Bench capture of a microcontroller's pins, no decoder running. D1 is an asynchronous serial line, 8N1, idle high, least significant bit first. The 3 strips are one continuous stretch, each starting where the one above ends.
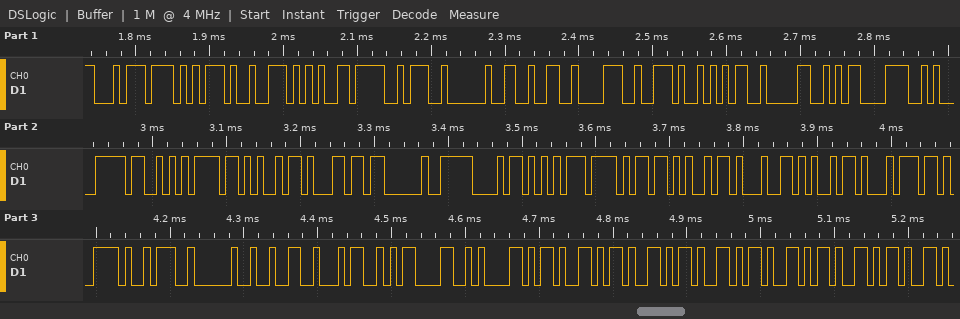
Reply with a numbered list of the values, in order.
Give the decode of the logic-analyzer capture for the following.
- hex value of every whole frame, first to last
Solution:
1. 74 75 72 65 3A 20 32 38 2E 35 30 0D 0A 53 6F 69 6C 20 68 75 6D 69 64 69 74 79 3A 20 32 34 0D 0A 2D 2D 2D 2D 2D 2D
